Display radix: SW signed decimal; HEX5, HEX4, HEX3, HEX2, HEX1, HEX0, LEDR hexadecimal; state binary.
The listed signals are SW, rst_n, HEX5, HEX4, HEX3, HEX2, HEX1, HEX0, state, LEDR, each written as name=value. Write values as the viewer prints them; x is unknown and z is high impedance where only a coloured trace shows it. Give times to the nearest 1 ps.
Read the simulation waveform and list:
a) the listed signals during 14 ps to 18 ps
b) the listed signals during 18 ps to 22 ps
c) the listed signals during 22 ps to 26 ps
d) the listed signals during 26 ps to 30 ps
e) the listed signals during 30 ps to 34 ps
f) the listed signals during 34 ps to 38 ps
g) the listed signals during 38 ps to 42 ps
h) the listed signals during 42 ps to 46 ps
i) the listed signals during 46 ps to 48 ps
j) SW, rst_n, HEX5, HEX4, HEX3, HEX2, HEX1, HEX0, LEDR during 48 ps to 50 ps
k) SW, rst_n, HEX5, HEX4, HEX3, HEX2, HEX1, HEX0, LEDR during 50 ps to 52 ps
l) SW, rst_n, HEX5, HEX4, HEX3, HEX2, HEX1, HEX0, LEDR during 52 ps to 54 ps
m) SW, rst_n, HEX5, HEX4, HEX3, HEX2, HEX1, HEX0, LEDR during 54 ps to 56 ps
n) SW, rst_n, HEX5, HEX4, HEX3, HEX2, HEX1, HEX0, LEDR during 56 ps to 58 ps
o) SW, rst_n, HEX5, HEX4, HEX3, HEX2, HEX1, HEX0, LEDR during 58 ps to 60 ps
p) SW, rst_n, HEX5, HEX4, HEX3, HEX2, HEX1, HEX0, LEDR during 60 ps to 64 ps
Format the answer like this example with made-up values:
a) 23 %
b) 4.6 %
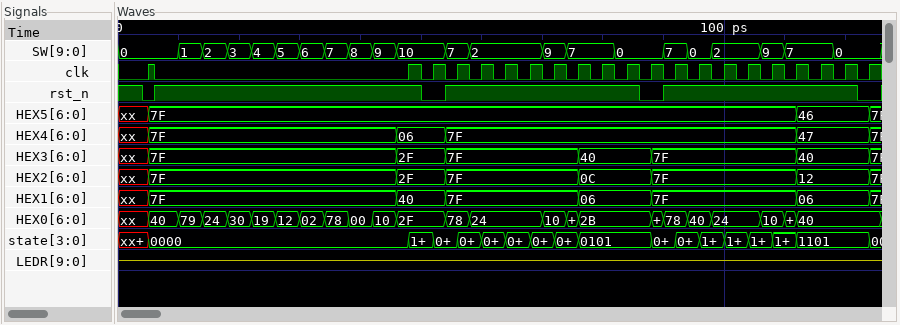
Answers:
a) SW=2, rst_n=1, HEX5=7F, HEX4=7F, HEX3=7F, HEX2=7F, HEX1=7F, HEX0=24, state=0000, LEDR=z
b) SW=3, rst_n=1, HEX5=7F, HEX4=7F, HEX3=7F, HEX2=7F, HEX1=7F, HEX0=30, state=0000, LEDR=z
c) SW=4, rst_n=1, HEX5=7F, HEX4=7F, HEX3=7F, HEX2=7F, HEX1=7F, HEX0=19, state=0000, LEDR=z
d) SW=5, rst_n=1, HEX5=7F, HEX4=7F, HEX3=7F, HEX2=7F, HEX1=7F, HEX0=12, state=0000, LEDR=z
e) SW=6, rst_n=1, HEX5=7F, HEX4=7F, HEX3=7F, HEX2=7F, HEX1=7F, HEX0=02, state=0000, LEDR=z
f) SW=7, rst_n=1, HEX5=7F, HEX4=7F, HEX3=7F, HEX2=7F, HEX1=7F, HEX0=78, state=0000, LEDR=z
g) SW=8, rst_n=1, HEX5=7F, HEX4=7F, HEX3=7F, HEX2=7F, HEX1=7F, HEX0=00, state=0000, LEDR=z
h) SW=9, rst_n=1, HEX5=7F, HEX4=7F, HEX3=7F, HEX2=7F, HEX1=7F, HEX0=10, state=0000, LEDR=z
i) SW=10, rst_n=1, HEX5=7F, HEX4=06, HEX3=2F, HEX2=2F, HEX1=40, HEX0=2F, state=0000, LEDR=z
j) SW=10, rst_n=1, HEX5=7F, HEX4=06, HEX3=2F, HEX2=2F, HEX1=40, HEX0=2F, LEDR=z
k) SW=10, rst_n=0, HEX5=7F, HEX4=06, HEX3=2F, HEX2=2F, HEX1=40, HEX0=2F, LEDR=z
l) SW=10, rst_n=0, HEX5=7F, HEX4=06, HEX3=2F, HEX2=2F, HEX1=40, HEX0=2F, LEDR=z
m) SW=7, rst_n=1, HEX5=7F, HEX4=7F, HEX3=7F, HEX2=7F, HEX1=7F, HEX0=78, LEDR=z
n) SW=7, rst_n=1, HEX5=7F, HEX4=7F, HEX3=7F, HEX2=7F, HEX1=7F, HEX0=78, LEDR=z
o) SW=2, rst_n=1, HEX5=7F, HEX4=7F, HEX3=7F, HEX2=7F, HEX1=7F, HEX0=24, LEDR=z
p) SW=2, rst_n=1, HEX5=7F, HEX4=7F, HEX3=7F, HEX2=7F, HEX1=7F, HEX0=24, LEDR=z
